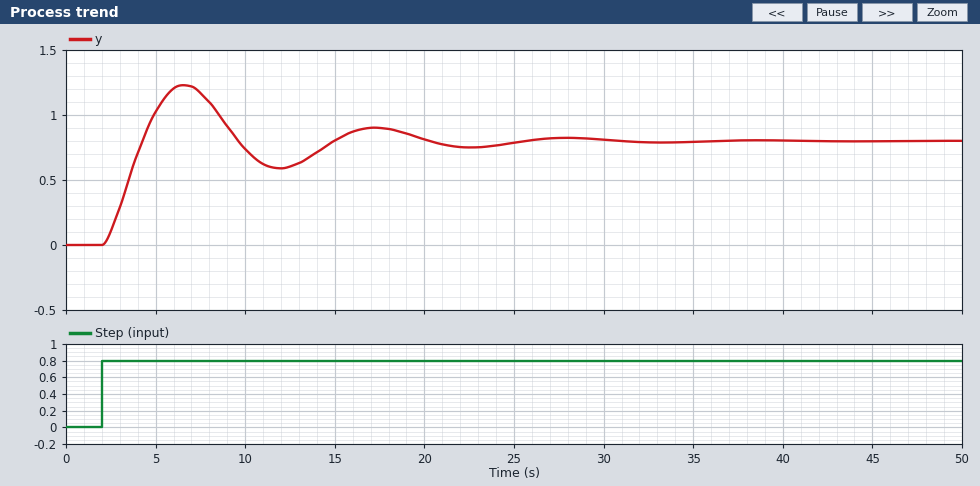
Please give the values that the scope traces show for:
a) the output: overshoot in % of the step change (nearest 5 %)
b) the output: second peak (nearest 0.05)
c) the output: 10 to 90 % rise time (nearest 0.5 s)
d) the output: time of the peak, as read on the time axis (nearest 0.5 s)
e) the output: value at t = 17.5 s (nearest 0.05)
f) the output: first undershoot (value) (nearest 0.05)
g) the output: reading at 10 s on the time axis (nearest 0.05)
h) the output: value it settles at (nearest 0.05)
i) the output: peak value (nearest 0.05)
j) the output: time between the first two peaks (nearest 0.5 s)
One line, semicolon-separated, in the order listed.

55 %; 0.90; 1.5 s; 6.5 s; 0.90; 0.60; 0.75; 0.80; 1.25; 10.5 s
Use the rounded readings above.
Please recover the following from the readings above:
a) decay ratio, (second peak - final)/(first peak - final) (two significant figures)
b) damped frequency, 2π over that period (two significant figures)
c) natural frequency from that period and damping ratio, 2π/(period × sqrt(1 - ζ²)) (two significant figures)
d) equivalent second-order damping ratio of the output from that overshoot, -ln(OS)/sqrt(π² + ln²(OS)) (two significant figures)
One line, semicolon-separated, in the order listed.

0.22; 0.60 rad/s; 0.61 rad/s; 0.19
